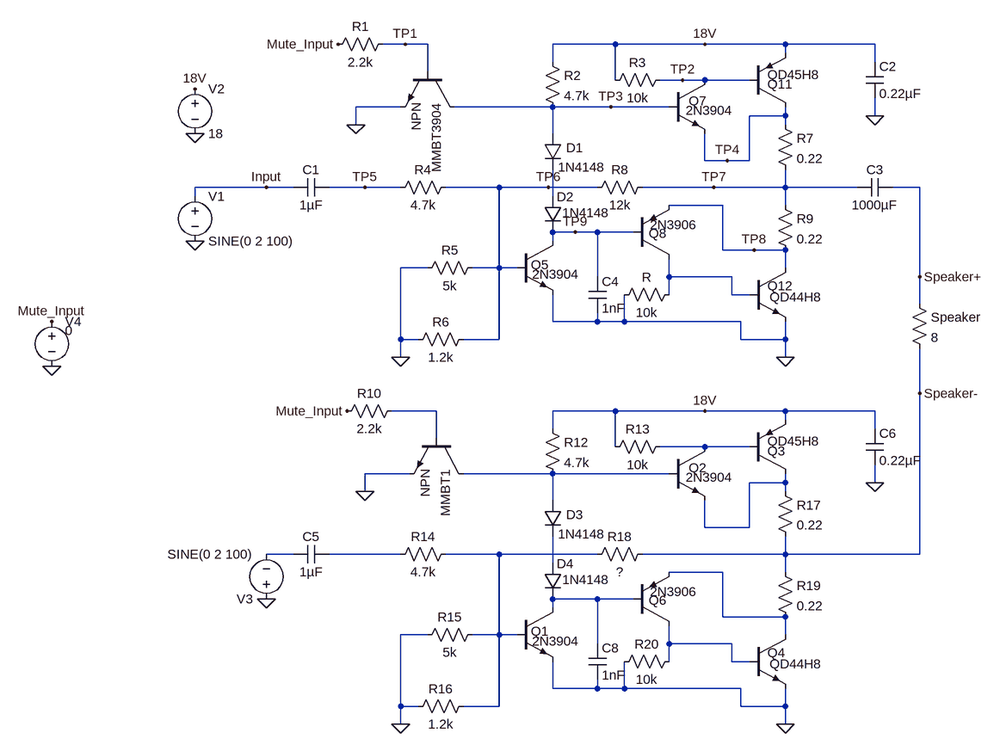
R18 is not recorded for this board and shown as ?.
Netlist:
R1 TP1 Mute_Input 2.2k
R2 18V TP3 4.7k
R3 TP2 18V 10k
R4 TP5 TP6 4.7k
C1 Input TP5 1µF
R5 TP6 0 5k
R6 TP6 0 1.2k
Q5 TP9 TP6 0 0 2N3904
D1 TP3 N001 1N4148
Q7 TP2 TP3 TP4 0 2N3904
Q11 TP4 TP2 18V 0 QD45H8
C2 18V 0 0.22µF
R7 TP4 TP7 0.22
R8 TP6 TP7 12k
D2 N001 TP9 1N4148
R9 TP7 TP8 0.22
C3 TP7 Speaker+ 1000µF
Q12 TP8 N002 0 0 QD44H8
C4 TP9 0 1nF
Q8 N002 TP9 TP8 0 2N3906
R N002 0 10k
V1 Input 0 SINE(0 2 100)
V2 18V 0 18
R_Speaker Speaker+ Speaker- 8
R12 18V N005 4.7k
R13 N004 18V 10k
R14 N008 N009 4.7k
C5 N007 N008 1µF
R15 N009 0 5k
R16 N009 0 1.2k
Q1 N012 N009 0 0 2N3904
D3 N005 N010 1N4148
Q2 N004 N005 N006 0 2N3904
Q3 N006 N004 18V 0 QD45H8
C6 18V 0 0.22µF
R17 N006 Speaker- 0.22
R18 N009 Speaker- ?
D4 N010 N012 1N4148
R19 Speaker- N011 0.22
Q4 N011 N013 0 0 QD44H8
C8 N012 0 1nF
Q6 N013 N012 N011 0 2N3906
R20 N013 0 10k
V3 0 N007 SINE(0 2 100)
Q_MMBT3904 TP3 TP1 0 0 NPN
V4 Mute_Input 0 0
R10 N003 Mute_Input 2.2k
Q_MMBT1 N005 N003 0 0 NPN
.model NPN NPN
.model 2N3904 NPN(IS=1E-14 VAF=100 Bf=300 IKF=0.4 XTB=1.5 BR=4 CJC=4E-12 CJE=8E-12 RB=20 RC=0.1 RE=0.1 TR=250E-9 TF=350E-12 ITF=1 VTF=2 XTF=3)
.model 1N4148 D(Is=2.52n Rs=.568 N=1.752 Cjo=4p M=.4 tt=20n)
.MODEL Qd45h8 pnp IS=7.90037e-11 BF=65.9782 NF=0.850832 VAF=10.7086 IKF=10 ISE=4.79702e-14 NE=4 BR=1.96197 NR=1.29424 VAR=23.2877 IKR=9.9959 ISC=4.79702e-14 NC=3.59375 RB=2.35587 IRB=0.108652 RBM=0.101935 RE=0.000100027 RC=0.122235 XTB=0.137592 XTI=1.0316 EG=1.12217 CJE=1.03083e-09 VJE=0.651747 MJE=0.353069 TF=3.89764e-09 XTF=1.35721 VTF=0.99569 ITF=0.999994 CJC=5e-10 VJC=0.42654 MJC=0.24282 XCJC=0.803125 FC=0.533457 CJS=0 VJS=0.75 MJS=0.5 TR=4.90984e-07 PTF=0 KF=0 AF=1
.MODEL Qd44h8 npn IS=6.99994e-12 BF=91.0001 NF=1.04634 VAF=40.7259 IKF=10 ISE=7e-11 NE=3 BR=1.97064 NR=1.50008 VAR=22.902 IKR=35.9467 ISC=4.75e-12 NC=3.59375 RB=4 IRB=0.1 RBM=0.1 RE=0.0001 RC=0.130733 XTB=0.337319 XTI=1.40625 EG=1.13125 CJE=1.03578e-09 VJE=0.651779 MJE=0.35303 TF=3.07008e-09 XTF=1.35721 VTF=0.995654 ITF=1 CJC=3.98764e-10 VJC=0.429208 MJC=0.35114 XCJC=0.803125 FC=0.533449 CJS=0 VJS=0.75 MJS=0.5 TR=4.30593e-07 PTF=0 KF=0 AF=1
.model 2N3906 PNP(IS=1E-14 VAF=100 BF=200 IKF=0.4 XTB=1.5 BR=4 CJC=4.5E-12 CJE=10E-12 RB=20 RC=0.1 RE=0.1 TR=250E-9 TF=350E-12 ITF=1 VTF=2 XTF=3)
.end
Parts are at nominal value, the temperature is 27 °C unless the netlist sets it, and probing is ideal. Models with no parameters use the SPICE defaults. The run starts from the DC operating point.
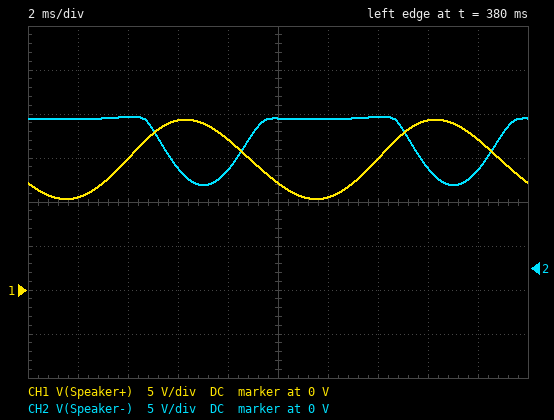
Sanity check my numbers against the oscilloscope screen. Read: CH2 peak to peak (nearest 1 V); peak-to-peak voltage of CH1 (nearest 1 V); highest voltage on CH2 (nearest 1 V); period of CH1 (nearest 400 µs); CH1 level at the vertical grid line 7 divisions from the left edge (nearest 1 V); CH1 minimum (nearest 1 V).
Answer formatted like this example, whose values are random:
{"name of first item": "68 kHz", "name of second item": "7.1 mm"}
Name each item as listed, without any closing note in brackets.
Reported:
{"CH2 peak to peak": "8 V", "peak-to-peak voltage of CH1": "9 V", "highest voltage on CH2": "17 V", "period of CH1": "10.0 ms", "CH1 level at the vertical grid line 7 divisions from the left edge": "15 V", "CH1 minimum": "10 V"}
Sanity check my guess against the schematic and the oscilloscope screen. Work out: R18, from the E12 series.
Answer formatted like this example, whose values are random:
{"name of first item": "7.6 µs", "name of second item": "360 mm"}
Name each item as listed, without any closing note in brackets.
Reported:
{"R18, from the E12 series": "27 kΩ"}
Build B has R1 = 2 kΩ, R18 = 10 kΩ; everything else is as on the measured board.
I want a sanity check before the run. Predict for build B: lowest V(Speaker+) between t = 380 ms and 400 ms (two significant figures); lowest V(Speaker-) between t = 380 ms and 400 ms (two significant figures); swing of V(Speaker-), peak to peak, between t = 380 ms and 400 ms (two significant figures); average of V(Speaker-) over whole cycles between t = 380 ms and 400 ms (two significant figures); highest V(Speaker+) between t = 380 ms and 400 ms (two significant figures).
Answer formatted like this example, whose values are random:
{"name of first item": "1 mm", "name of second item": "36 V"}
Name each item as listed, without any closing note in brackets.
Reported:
{"lowest V(Speaker+) between t = 380 ms and 400 ms": "3.2 V", "lowest V(Speaker-) between t = 380 ms and 400 ms": "3.8 V", "swing of V(Speaker-), peak to peak, between t = 380 ms and 400 ms": "7.6 V", "average of V(Speaker-) over whole cycles between t = 380 ms and 400 ms": "7.7 V", "highest V(Speaker+) between t = 380 ms and 400 ms": "12 V"}
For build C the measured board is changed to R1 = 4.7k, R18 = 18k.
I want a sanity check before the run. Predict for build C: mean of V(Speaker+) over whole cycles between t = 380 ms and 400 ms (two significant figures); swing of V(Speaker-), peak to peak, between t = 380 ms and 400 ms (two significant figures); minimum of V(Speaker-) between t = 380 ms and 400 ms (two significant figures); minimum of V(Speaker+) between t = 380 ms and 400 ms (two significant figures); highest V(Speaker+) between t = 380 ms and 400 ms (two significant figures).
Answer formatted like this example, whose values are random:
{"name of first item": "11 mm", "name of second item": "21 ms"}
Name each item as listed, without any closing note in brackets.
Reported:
{"mean of V(Speaker+) over whole cycles between t = 380 ms and 400 ms": "12 V", "swing of V(Speaker-), peak to peak, between t = 380 ms and 400 ms": "10 V", "minimum of V(Speaker-) between t = 380 ms and 400 ms": "6.4 V", "minimum of V(Speaker+) between t = 380 ms and 400 ms": "7.8 V", "highest V(Speaker+) between t = 380 ms and 400 ms": "17 V"}
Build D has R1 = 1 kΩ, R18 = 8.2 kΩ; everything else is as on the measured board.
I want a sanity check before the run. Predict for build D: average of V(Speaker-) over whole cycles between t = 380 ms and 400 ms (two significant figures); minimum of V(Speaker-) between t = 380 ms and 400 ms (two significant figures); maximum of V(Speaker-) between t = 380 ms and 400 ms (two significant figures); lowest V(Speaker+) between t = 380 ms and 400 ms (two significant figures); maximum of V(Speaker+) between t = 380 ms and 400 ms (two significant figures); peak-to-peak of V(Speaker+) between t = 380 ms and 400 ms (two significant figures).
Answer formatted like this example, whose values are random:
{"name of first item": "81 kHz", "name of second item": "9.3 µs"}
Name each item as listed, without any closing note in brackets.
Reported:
{"average of V(Speaker-) over whole cycles between t = 380 ms and 400 ms": "6.5 V", "minimum of V(Speaker-) between t = 380 ms and 400 ms": "3.3 V", "maximum of V(Speaker-) between t = 380 ms and 400 ms": "9.6 V", "lowest V(Speaker+) between t = 380 ms and 400 ms": "2.0 V", "maximum of V(Speaker+) between t = 380 ms and 400 ms": "11 V", "peak-to-peak of V(Speaker+) between t = 380 ms and 400 ms": "8.9 V"}
